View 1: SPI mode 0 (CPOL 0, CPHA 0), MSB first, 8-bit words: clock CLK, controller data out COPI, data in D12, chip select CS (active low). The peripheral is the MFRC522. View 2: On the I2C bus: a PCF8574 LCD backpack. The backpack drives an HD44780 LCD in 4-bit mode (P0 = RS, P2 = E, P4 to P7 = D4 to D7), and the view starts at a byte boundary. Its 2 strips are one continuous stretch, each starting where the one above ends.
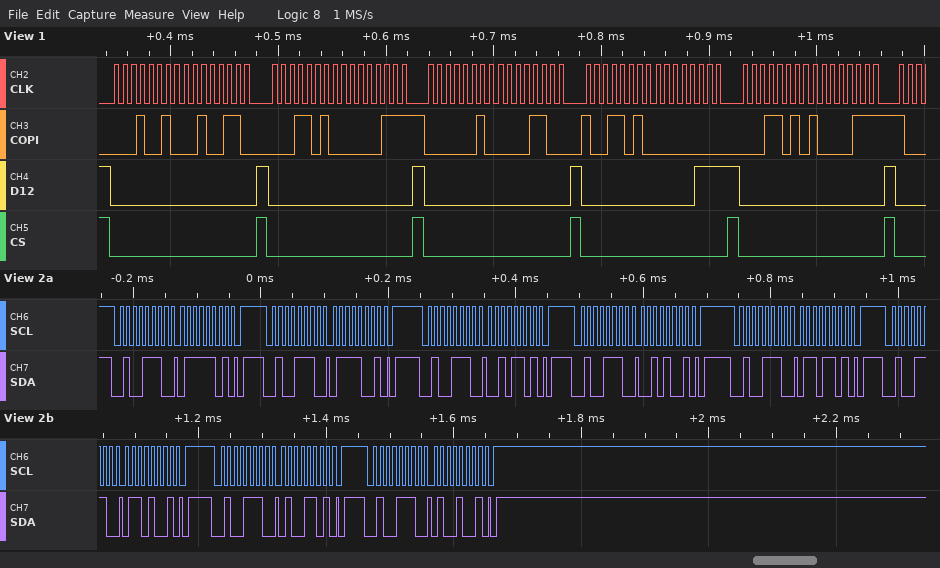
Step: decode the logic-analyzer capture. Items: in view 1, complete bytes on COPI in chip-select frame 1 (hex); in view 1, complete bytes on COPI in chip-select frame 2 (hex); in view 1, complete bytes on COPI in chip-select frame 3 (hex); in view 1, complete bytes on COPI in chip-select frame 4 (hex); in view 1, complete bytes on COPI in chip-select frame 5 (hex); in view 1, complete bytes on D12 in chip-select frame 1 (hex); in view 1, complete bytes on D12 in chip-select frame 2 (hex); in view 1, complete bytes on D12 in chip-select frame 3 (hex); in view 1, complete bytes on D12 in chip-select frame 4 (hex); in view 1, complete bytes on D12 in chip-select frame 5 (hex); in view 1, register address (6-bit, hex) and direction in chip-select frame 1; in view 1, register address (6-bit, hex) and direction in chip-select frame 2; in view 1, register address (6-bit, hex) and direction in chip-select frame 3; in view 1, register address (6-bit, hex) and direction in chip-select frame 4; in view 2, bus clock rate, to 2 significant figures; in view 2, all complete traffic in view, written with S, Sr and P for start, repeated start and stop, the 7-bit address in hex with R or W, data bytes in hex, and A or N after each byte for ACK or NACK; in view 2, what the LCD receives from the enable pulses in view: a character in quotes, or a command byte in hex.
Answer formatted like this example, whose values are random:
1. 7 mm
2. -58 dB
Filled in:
1. 12 26
2. 1A 07
3. 02 0C
4. 9A 00
5. 1A 87
6. 00 00
7. 00 00
8. 00 00
9. 00 07
10. 00 00
11. 0x09 write
12. 0x0D write
13. 0x01 write
14. 0x0D read
15. 100 kHz
16. S 27W A 7D A P S 27W A 79 A P S 27W A 2D A P S 27W A 29 A P S 27W A 6D A P S 27W A 69 A P S 27W A 4D A P S 27W A 49 A P
17. 'r' 'd'
